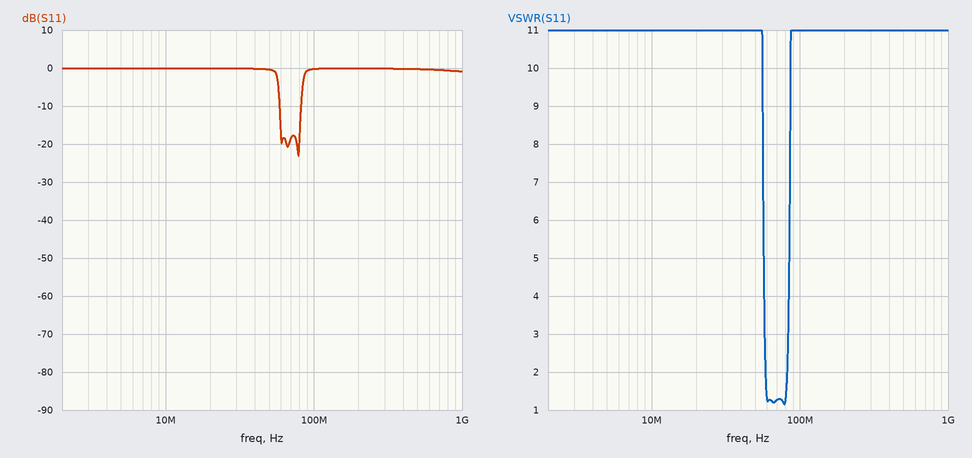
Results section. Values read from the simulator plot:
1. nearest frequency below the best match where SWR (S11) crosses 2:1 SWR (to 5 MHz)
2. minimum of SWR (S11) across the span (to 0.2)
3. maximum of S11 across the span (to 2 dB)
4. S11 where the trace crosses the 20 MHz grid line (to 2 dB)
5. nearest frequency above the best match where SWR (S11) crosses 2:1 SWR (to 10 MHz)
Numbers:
60 MHz
1.2
0 dB
0 dB
80 MHz
